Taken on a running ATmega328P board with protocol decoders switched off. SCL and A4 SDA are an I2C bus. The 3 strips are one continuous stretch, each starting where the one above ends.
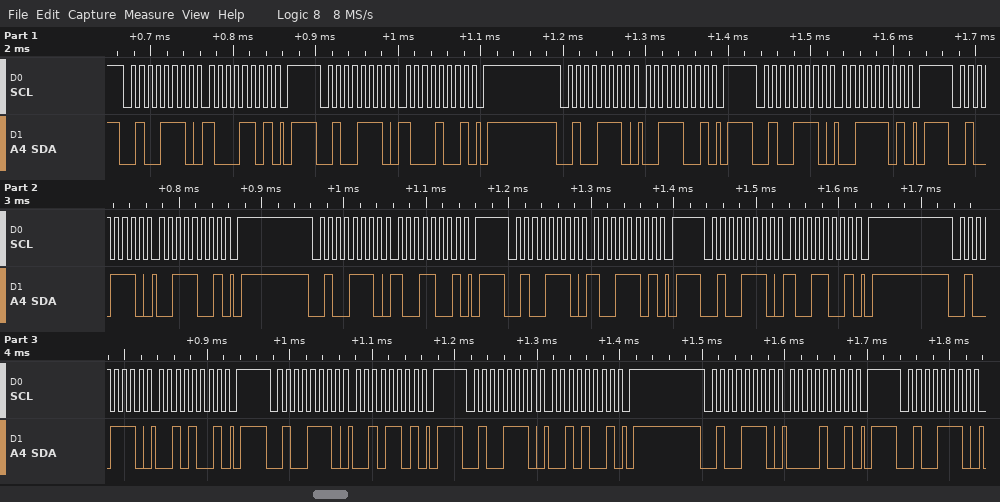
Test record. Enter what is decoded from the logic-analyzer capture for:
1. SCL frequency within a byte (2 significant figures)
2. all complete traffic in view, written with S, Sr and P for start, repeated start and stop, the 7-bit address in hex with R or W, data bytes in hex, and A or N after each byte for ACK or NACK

100 kHz
S 27W A 8D A P S 27W A 89 A P S 27W A 39 A P S 27W A 3D A P S 27W A 39 A P S 27W A 99 A P S 27W A 9D A P S 27W A 99 A P S 27W A 29 A P S 27W A 2D A P S 27W A 29 A P S 27W A 09 A P S 27W A
